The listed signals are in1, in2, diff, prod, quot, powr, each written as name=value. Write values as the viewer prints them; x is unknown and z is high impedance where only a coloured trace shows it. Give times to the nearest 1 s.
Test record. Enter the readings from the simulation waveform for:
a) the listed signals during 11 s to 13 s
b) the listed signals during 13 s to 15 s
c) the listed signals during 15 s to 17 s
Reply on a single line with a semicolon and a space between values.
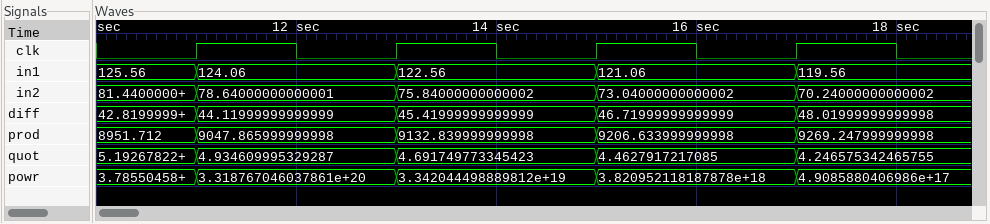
in1=124.06, in2=78.64000000000001, diff=44.11999999999999, prod=9047.865999999998, quot=4.934609995329287, powr=3.318767046037861e+20; in1=122.56, in2=75.84000000000002, diff=45.41999999999999, prod=9132.839999999998, quot=4.691749773345423, powr=3.342044498889812e+19; in1=121.06, in2=73.04000000000002, diff=46.71999999999999, prod=9206.633999999998, quot=4.4627917217085, powr=3.820952118187878e+18
